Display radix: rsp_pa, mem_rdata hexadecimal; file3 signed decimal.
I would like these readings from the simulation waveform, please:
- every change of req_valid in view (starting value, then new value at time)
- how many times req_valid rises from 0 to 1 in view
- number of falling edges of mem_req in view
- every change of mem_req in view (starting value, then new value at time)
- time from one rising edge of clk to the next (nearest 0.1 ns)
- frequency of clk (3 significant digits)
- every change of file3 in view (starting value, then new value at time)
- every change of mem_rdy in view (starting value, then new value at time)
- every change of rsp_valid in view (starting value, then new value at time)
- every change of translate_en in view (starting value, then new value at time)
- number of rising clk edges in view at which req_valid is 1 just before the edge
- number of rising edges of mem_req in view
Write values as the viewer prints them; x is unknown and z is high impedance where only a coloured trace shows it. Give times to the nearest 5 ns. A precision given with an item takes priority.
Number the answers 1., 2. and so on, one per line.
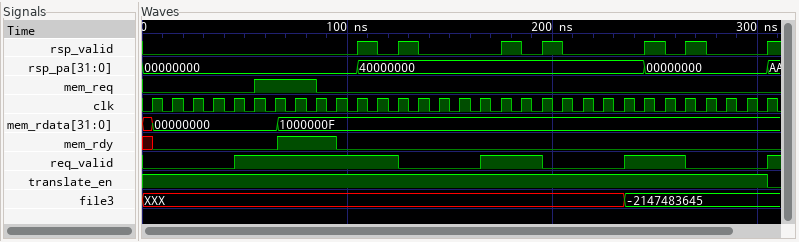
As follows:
1. 0, 1 at 45 ns, 0 at 125 ns, 1 at 165 ns, 0 at 195 ns, 1 at 235 ns, 0 at 265 ns, 1 at 305 ns
2. 4
3. 1
4. 0, 1 at 55 ns, 0 at 85 ns
5. 10 ns
6. 100 MHz
7. XXX, -2147483645 at 235 ns
8. x, 0 at 5 ns, 1 at 65 ns, 0 at 95 ns
9. 0, 1 at 105 ns, 0 at 115 ns, 1 at 125 ns, 0 at 135 ns, 1 at 175 ns, 0 at 185 ns, 1 at 195 ns, 0 at 205 ns, 1 at 245 ns, 0 at 255 ns, 1 at 265 ns, 0 at 275 ns, 1 at 305 ns
10. 1, 0 at 305 ns
11. 14
12. 1
